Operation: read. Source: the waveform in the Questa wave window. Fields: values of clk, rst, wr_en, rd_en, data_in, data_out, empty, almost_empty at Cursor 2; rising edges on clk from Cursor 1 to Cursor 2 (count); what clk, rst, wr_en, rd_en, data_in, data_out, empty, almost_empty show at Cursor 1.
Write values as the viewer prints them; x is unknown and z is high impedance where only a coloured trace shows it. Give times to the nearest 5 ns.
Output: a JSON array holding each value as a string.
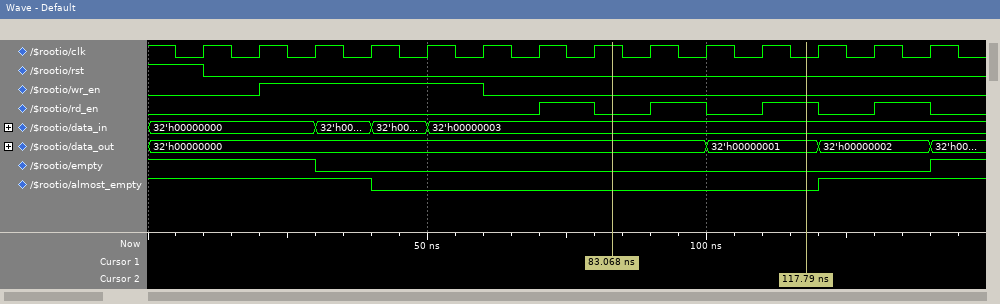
["clk=0, rst=0, wr_en=0, rd_en=1, data_in=32'h00000003, data_out=32'h00000001, empty=0, almost_empty=0", "3", "clk=1, rst=0, wr_en=0, rd_en=0, data_in=32'h00000003, data_out=32'h00000000, empty=0, almost_empty=0"]
